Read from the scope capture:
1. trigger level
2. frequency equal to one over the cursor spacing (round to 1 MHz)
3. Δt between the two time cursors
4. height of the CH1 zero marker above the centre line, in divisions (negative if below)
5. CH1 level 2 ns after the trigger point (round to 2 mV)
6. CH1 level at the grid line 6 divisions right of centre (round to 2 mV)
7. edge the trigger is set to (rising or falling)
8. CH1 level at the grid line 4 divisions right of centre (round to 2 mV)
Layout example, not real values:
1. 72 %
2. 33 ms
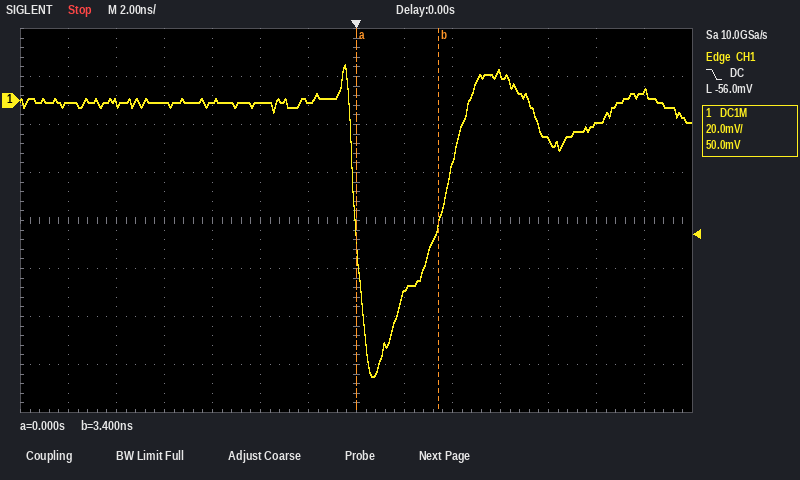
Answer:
1. -56.0 mV
2. 294 MHz
3. 3.4 ns
4. +2.5 div
5. -80 mV
6. 4 mV
7. falling
8. -16 mV
